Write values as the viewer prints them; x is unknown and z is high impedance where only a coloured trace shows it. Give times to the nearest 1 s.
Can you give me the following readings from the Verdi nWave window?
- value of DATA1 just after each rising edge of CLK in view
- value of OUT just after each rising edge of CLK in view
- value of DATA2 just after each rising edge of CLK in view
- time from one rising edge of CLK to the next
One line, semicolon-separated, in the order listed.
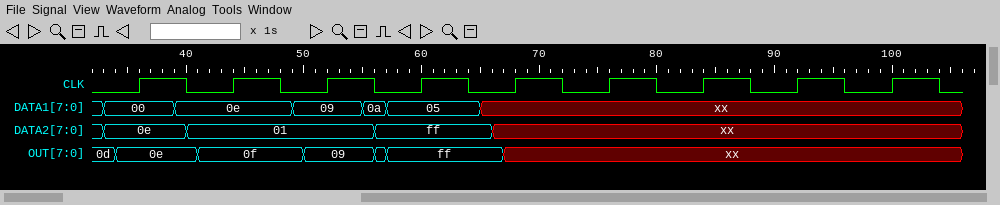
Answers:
00, 0e, 09, 05, xx, xx, xx, xx, xx; 0e, 0f, 09, ff, xx, xx, xx, xx, xx; 0e, 01, 01, ff, xx, xx, xx, xx, xx; 8 s
